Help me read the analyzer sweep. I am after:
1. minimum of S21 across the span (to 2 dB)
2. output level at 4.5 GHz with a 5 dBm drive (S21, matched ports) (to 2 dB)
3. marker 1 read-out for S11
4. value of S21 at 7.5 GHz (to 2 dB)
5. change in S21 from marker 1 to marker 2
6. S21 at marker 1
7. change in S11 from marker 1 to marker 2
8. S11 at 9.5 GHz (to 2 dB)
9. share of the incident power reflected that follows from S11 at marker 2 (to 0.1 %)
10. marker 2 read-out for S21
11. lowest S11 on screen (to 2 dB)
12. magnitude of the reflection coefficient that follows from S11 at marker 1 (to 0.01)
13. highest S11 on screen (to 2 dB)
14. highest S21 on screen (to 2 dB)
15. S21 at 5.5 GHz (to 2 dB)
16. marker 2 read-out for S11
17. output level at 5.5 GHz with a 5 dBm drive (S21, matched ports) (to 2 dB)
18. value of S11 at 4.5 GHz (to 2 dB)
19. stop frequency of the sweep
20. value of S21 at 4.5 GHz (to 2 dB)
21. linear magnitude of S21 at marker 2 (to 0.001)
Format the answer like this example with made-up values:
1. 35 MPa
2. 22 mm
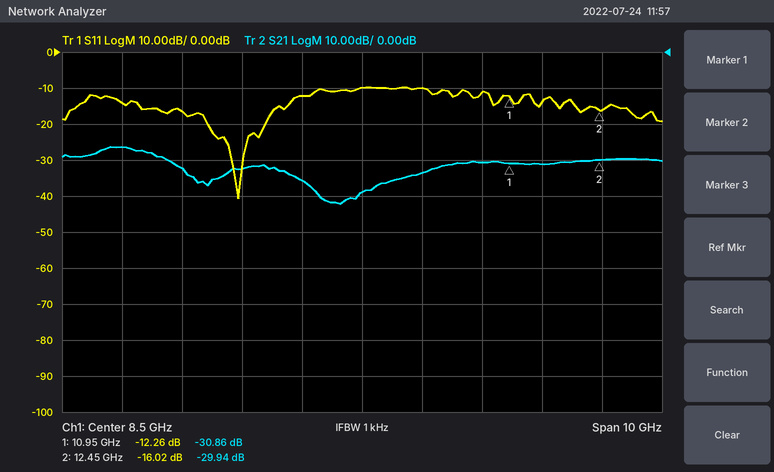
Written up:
1. -42 dB
2. -22 dBm
3. -12.26 dB
4. -36 dB
5. 0.92 dB
6. -30.86 dB
7. -3.76 dB
8. -10 dB
9. 2.5 %
10. -29.94 dB
11. -40 dB
12. 0.24
13. -10 dB
14. -26 dB
15. -32 dB
16. -16.02 dB
17. -28 dBm
18. -14 dB
19. 13.5 GHz
20. -26 dB
21. 0.032
